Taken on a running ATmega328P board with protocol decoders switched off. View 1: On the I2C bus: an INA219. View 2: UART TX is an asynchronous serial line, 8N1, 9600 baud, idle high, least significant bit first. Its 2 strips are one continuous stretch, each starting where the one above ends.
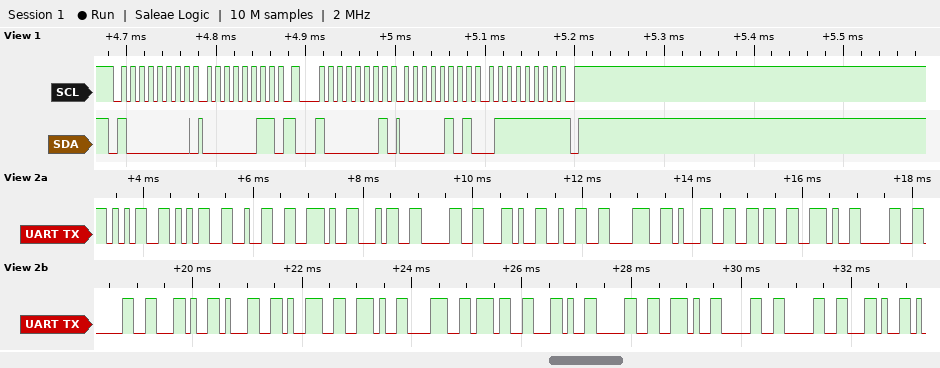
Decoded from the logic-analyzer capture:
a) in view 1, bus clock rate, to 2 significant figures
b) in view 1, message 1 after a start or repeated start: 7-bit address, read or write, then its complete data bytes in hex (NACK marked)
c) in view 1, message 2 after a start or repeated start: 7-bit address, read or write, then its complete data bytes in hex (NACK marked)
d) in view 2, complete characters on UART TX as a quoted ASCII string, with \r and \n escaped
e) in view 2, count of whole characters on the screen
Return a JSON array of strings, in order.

["100 kHz", "0x40 write: 03", "0x40 read: 05 7F NACK", "\"552.40,2816.00,19.87,0.00,\"", "26"]
